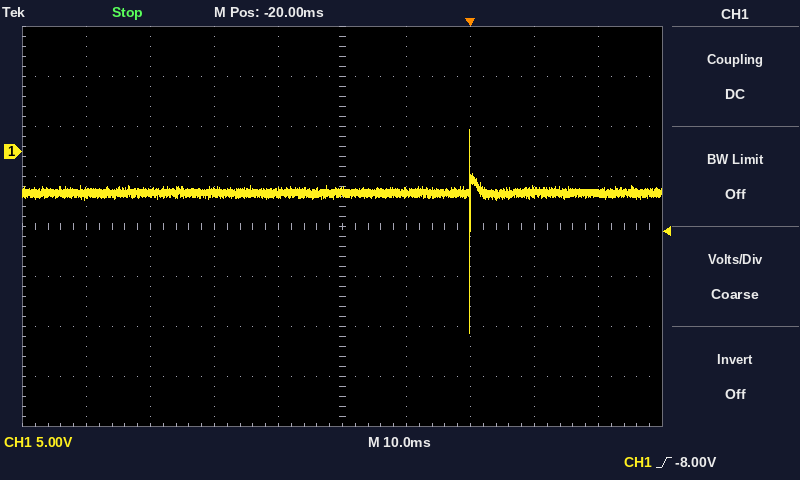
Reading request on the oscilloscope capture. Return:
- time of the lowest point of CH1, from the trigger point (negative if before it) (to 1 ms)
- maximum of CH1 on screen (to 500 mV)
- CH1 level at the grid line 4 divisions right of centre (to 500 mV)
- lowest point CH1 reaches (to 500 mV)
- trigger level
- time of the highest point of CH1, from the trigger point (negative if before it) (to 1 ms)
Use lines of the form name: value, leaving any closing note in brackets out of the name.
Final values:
time of the lowest point of CH1, from the trigger point (negative if before it): 0 ms
maximum of CH1 on screen: 2.0 V
CH1 level at the grid line 4 divisions right of centre: -4.0 V
lowest point CH1 reaches: -18.0 V
trigger level: -8.00 V
time of the highest point of CH1, from the trigger point (negative if before it): 0 ms
